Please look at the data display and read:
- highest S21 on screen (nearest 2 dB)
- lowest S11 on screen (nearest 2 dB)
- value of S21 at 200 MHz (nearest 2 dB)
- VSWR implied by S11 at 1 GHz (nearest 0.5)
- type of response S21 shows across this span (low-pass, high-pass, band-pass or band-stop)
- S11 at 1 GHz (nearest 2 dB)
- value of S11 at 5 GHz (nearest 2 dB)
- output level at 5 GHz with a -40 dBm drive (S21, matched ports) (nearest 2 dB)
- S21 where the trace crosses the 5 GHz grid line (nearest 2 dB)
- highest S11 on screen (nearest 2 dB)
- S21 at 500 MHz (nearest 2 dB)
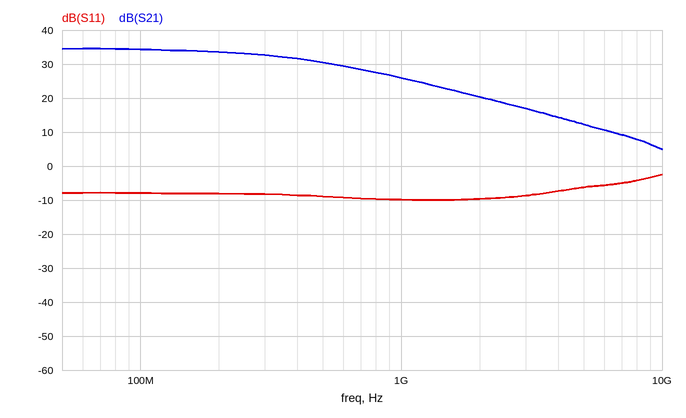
34 dB
-10 dB
34 dB
2.0
low-pass
-10 dB
-6 dB
-28 dBm
12 dB
-2 dB
30 dB
